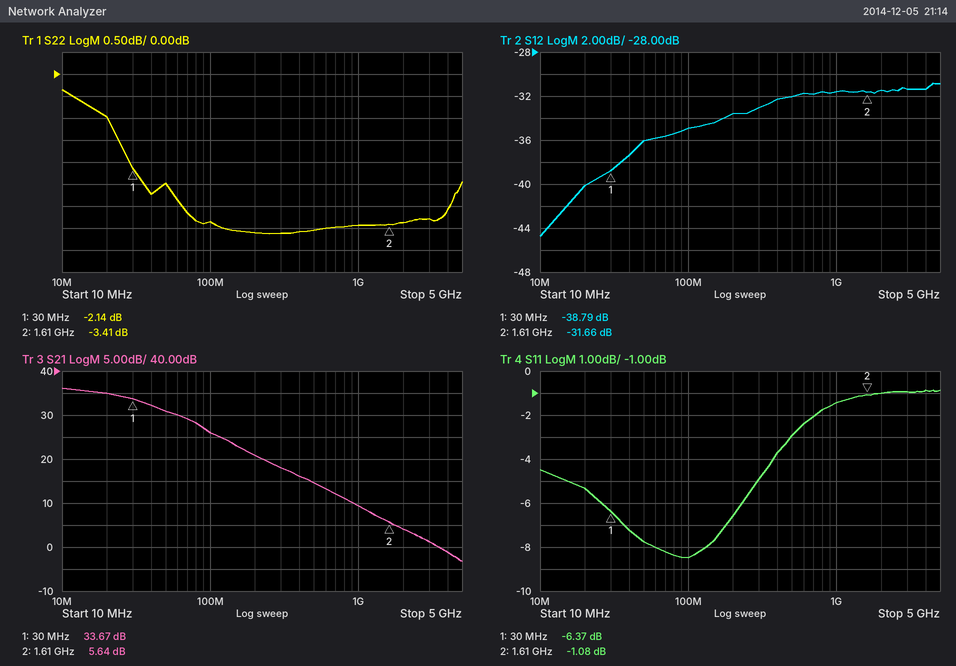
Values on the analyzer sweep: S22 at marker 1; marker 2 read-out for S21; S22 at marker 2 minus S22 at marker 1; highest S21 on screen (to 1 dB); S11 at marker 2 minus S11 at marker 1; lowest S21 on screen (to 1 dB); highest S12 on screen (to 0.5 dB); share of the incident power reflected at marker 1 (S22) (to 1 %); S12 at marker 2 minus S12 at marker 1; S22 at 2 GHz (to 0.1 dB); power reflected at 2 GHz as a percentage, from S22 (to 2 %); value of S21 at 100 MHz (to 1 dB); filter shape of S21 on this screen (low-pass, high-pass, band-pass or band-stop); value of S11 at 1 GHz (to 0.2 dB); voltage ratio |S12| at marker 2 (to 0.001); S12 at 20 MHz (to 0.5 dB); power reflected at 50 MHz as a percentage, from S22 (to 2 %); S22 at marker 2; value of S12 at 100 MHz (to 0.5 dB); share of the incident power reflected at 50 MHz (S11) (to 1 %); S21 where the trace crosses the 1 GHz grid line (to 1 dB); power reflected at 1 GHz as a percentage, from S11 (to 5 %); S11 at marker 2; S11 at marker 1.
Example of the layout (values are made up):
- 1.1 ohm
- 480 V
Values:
- -2.14 dB
- 5.64 dB
- -1.27 dB
- 36 dB
- 5.29 dB
- -3 dB
- -31.0 dB
- 61 %
- 7.13 dB
- -3.4 dB
- 46 %
- 26 dB
- low-pass
- -1.4 dB
- 0.026
- -40.0 dB
- 56 %
- -3.41 dB
- -35.0 dB
- 17 %
- 9 dB
- 70 %
- -1.08 dB
- -6.37 dB
